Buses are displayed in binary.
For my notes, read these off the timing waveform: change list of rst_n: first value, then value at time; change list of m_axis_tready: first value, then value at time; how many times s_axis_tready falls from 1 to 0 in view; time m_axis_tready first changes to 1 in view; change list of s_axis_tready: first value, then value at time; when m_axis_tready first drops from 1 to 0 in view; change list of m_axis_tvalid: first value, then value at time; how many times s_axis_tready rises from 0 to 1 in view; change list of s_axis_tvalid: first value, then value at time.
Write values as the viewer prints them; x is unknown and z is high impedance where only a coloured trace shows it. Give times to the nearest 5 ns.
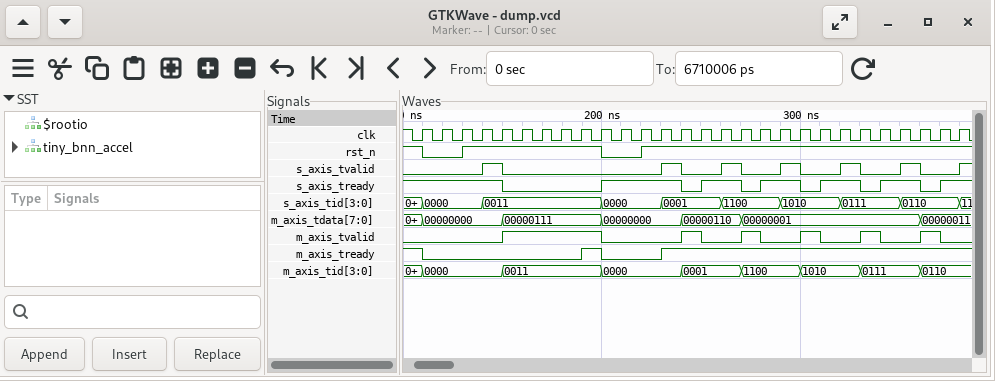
1, 0 at 110 ns, 1 at 130 ns, 0 at 200 ns, 1 at 220 ns
1, 0 at 110 ns, 1 at 190 ns, 0 at 200 ns, 1 at 230 ns
6
190 ns
1, 0 at 150 ns, 1 at 200 ns, 0 at 240 ns, 1 at 250 ns, 0 at 270 ns, 1 at 280 ns, 0 at 300 ns, 1 at 310 ns, 0 at 330 ns, 1 at 340 ns, 0 at 360 ns, 1 at 370 ns
110 ns
0, 1 at 150 ns, 0 at 200 ns, 1 at 240 ns, 0 at 250 ns, 1 at 270 ns, 0 at 280 ns, 1 at 300 ns, 0 at 310 ns, 1 at 330 ns, 0 at 340 ns, 1 at 360 ns, 0 at 370 ns
6
0, 1 at 140 ns, 0 at 150 ns, 1 at 230 ns, 0 at 240 ns, 1 at 260 ns, 0 at 270 ns, 1 at 290 ns, 0 at 300 ns, 1 at 320 ns, 0 at 330 ns, 1 at 350 ns, 0 at 360 ns, 1 at 380 ns
